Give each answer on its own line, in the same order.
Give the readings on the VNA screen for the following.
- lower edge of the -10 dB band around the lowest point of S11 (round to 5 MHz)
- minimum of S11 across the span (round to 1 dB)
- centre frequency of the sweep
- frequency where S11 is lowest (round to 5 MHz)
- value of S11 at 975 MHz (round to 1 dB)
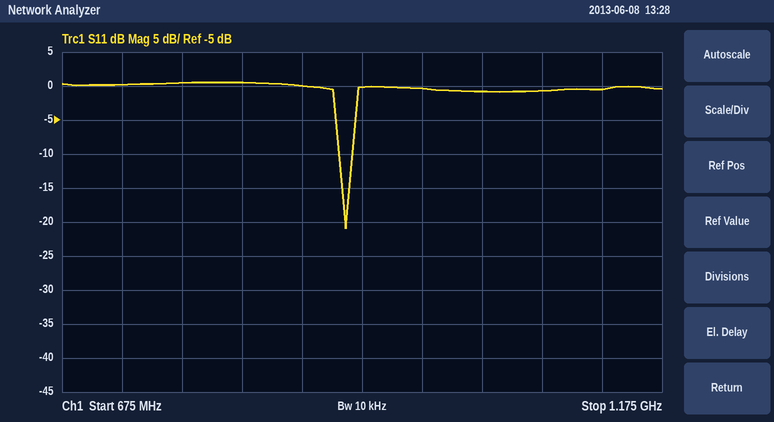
905 MHz
-21 dB
925 MHz
910 MHz
0 dB
